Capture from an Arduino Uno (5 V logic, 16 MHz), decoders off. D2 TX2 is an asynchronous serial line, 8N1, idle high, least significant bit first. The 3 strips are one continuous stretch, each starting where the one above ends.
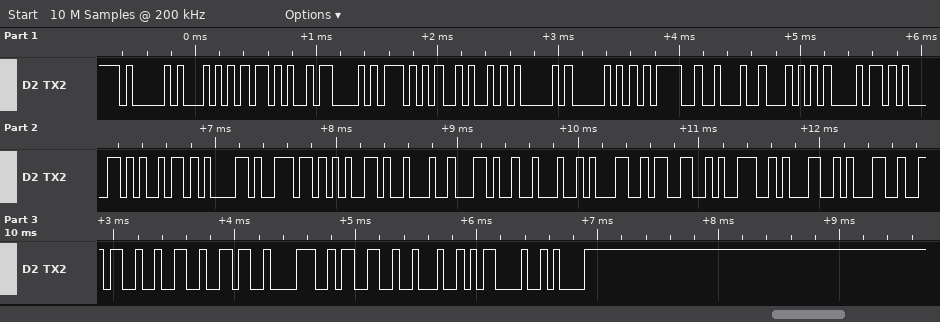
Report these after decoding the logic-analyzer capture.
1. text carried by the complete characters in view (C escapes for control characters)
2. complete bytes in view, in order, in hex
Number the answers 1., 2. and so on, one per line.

1. "AT+CWJAP=\"Thaiane\",\"1391162683\"\r\n"
2. 41 54 2B 43 57 4A 41 50 3D 22 54 68 61 69 61 6E 65 22 2C 22 31 33 39 31 31 36 32 36 38 33 22 0D 0A
